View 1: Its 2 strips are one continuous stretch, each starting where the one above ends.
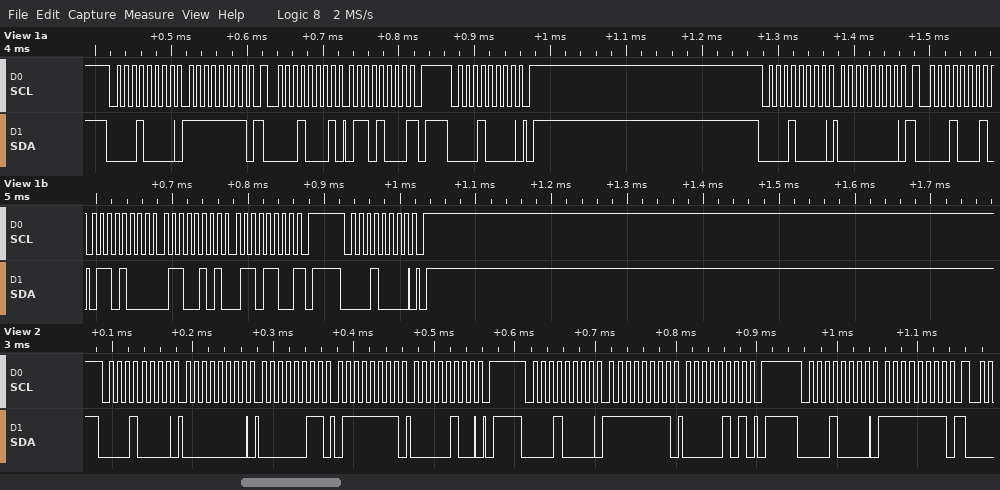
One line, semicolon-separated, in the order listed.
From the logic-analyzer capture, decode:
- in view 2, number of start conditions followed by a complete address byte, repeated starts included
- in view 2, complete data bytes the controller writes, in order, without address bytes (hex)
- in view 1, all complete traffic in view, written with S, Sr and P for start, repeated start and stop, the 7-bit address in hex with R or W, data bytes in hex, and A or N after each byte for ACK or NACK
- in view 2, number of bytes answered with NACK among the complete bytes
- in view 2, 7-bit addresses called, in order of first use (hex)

3; 00 03 7F 04 FF 05 FF; S 08W A FF A Sr 08R A 68 N P S 08W A P S 08W A 00 A Sr 08R A 68 A 65 A 6C N P S 08W A P; 0; 0x08
